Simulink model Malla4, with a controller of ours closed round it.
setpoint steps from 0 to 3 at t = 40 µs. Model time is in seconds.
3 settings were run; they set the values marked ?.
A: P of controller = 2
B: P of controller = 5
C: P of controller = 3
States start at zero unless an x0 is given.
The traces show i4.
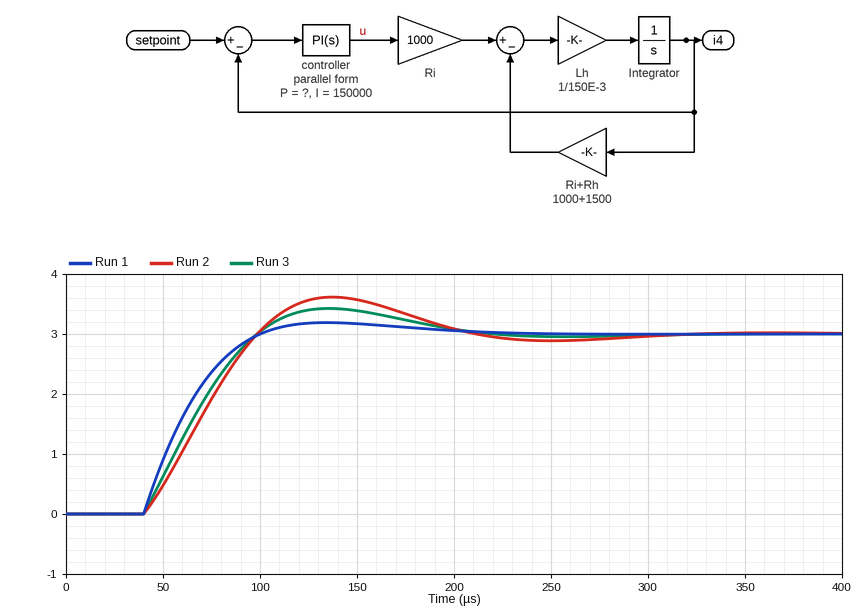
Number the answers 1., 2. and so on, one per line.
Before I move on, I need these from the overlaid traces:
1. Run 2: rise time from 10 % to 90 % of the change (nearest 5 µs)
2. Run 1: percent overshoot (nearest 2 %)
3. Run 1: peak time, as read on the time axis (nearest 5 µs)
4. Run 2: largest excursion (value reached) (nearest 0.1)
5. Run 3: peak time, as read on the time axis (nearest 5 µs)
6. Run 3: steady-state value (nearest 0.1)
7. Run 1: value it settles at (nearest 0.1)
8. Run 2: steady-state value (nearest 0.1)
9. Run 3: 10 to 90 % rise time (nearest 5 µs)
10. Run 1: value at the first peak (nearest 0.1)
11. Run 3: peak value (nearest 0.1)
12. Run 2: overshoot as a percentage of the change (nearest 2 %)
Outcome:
1. 45 µs
2. 6 %
3. 135 µs
4. 3.6
5. 135 µs
6. 3.0
7. 3.0
8. 3.0
9. 45 µs
10. 3.2
11. 3.4
12. 20 %
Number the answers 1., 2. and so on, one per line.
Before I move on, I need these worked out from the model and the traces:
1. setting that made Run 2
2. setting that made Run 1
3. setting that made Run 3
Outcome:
1. A
2. B
3. C
